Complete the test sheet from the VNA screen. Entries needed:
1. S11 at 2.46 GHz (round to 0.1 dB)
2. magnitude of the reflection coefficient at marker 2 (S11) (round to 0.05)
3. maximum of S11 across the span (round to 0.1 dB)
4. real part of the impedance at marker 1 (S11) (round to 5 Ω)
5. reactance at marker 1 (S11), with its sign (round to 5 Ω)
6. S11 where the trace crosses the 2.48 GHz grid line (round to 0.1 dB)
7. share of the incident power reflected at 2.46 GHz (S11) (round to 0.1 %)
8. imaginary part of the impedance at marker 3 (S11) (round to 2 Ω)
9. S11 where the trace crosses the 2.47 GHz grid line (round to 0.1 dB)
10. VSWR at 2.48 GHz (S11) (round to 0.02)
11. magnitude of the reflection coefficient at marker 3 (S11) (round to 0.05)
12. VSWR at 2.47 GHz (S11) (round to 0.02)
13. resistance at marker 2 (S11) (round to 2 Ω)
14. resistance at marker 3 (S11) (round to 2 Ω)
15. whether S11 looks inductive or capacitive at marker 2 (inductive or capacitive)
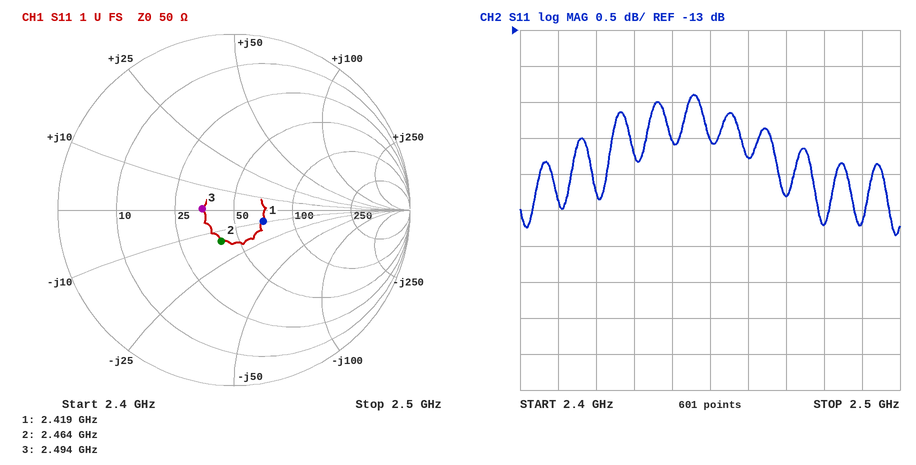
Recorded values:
-14.8 dB
0.20
-13.9 dB
70 Ω
-10 Ω
-15.7 dB
3.3 %
0 Ω
-15.3 dB
1.40
0.20
1.42
40 Ω
34 Ω
capacitive
